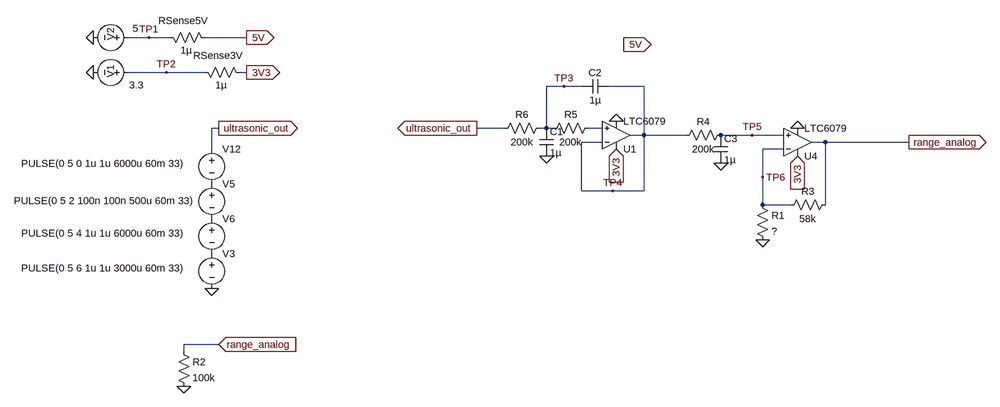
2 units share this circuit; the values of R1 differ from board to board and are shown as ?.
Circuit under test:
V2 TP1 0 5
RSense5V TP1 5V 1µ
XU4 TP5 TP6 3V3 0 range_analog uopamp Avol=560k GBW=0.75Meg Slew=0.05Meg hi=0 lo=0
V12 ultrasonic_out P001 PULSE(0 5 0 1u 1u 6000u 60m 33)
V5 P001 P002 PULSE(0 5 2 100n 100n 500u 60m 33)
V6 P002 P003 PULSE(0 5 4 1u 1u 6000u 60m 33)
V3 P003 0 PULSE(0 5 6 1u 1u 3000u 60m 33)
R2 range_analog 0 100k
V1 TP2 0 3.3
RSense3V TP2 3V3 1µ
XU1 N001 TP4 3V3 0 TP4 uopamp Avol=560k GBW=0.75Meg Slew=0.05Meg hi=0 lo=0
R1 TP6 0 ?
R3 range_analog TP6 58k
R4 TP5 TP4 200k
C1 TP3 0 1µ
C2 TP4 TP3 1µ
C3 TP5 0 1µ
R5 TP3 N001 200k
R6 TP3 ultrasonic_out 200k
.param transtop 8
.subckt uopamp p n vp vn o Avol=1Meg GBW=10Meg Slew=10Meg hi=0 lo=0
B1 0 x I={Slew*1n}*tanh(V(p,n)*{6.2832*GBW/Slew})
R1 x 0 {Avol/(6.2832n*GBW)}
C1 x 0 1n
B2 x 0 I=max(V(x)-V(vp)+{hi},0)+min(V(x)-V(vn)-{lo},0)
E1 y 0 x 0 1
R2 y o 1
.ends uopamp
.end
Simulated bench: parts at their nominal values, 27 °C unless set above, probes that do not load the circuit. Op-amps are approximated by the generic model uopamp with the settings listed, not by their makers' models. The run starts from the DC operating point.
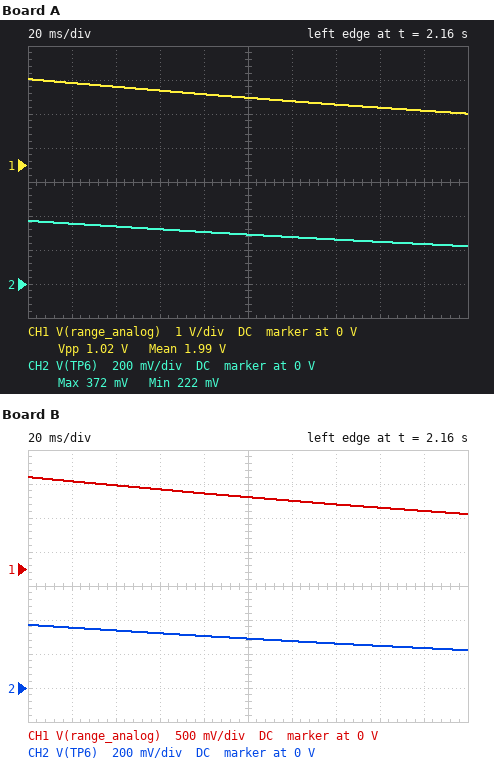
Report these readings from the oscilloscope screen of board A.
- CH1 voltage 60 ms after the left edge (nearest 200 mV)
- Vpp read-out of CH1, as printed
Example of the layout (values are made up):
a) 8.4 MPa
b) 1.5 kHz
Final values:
a) 2.2 V
b) 1.02 V
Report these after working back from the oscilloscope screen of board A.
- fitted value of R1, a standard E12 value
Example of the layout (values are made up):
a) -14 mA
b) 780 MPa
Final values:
a) 10 kΩ
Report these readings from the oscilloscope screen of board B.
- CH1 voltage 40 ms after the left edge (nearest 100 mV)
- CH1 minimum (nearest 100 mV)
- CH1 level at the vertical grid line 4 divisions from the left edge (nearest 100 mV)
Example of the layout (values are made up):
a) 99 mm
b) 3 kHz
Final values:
a) 1.2 V
b) 800 mV
c) 1.1 V
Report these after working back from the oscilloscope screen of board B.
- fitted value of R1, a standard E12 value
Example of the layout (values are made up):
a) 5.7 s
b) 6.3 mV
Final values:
a) 22 kΩ
